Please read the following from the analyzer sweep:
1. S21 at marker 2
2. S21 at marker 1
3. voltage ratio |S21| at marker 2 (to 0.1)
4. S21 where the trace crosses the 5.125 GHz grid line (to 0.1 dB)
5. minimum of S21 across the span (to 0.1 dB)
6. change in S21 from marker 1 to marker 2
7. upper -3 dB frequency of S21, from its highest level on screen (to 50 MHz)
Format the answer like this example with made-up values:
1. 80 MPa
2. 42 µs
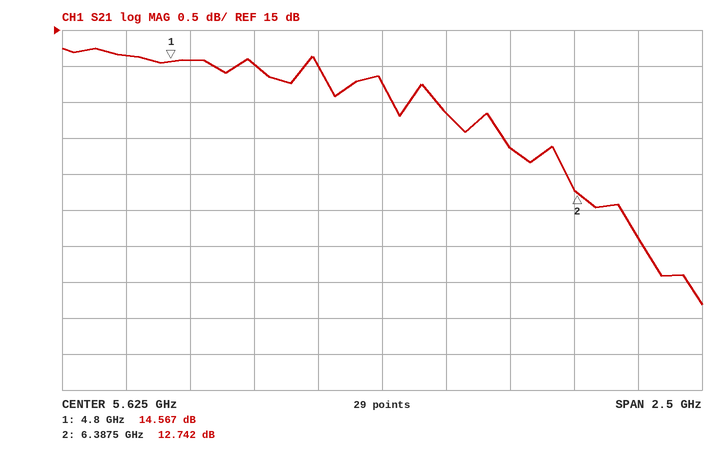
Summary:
1. 12.742 dB
2. 14.567 dB
3. 4.3
4. 14.5 dB
5. 11.2 dB
6. -1.825 dB
7. 6.70 GHz
